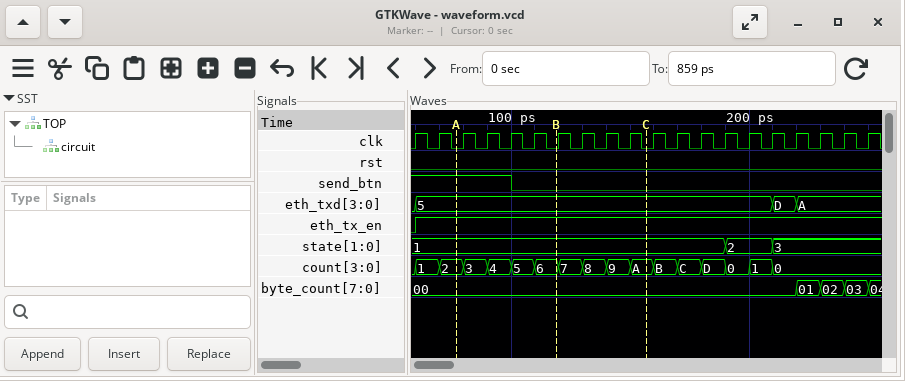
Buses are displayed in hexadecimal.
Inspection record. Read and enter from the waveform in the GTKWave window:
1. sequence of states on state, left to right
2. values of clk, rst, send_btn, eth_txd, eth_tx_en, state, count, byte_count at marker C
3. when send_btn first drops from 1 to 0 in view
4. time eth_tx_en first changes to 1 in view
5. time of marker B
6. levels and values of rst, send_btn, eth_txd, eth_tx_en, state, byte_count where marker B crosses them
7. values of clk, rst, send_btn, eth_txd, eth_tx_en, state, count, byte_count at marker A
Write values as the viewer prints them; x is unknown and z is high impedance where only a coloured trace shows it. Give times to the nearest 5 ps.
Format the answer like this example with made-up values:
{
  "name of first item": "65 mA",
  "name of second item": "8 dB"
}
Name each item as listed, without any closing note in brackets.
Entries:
{
  "sequence of states on state, left to right": "1, 2, 3",
  "values of clk, rst, send_btn, eth_txd, eth_tx_en, state, count, byte_count at marker C": "clk=0, rst=0, send_btn=0, eth_txd=5, eth_tx_en=1, state=1, count=A, byte_count=00",
  "when send_btn first drops from 1 to 0 in view": "100 ps",
  "time eth_tx_en first changes to 1 in view": "60 ps",
  "time of marker B": "120 ps",
  "levels and values of rst, send_btn, eth_txd, eth_tx_en, state, byte_count where marker B crosses them": "rst=0, send_btn=0, eth_txd=5, eth_tx_en=1, state=1, byte_count=00",
  "values of clk, rst, send_btn, eth_txd, eth_tx_en, state, count, byte_count at marker A": "clk=0, rst=0, send_btn=1, eth_txd=5, eth_tx_en=1, state=1, count=2, byte_count=00"
}
